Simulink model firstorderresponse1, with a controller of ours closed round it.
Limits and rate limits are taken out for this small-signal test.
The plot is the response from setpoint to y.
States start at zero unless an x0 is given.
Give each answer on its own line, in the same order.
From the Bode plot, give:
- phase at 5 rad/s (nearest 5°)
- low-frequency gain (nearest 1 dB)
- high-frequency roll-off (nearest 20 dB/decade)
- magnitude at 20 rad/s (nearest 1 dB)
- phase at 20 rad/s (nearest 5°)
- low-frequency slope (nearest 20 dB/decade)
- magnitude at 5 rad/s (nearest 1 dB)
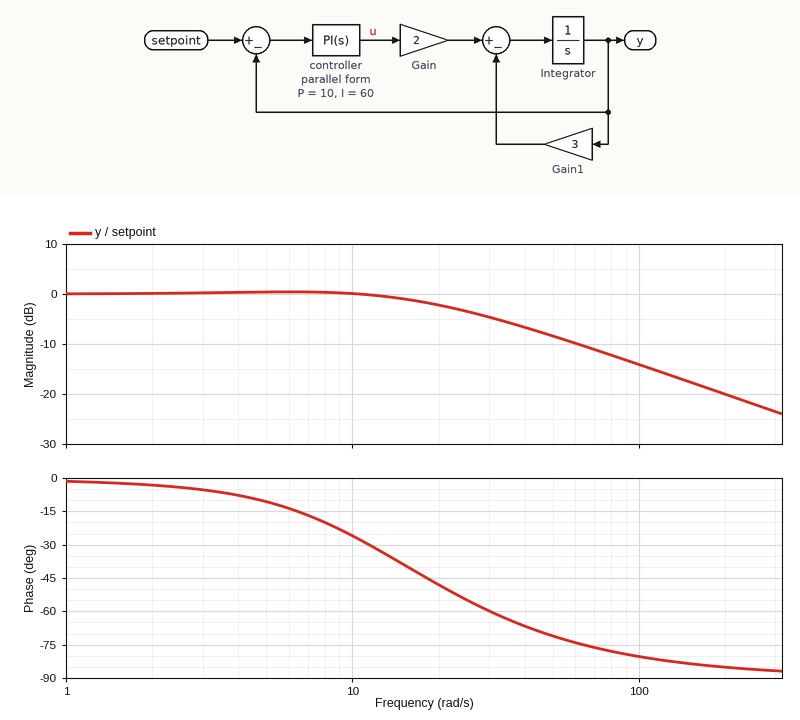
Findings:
-10°
0 dB
-20 dB/decade
-2 dB
-50°
0 dB/decade
0 dB
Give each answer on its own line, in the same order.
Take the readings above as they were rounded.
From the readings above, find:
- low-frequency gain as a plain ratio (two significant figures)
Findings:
1.0
